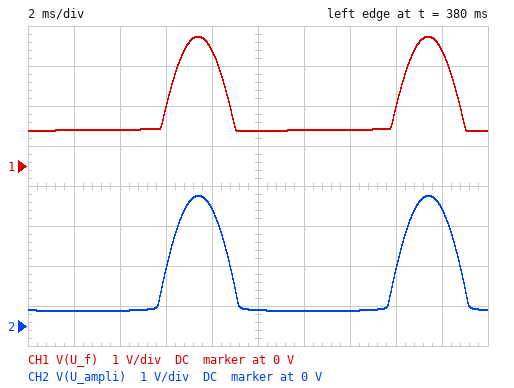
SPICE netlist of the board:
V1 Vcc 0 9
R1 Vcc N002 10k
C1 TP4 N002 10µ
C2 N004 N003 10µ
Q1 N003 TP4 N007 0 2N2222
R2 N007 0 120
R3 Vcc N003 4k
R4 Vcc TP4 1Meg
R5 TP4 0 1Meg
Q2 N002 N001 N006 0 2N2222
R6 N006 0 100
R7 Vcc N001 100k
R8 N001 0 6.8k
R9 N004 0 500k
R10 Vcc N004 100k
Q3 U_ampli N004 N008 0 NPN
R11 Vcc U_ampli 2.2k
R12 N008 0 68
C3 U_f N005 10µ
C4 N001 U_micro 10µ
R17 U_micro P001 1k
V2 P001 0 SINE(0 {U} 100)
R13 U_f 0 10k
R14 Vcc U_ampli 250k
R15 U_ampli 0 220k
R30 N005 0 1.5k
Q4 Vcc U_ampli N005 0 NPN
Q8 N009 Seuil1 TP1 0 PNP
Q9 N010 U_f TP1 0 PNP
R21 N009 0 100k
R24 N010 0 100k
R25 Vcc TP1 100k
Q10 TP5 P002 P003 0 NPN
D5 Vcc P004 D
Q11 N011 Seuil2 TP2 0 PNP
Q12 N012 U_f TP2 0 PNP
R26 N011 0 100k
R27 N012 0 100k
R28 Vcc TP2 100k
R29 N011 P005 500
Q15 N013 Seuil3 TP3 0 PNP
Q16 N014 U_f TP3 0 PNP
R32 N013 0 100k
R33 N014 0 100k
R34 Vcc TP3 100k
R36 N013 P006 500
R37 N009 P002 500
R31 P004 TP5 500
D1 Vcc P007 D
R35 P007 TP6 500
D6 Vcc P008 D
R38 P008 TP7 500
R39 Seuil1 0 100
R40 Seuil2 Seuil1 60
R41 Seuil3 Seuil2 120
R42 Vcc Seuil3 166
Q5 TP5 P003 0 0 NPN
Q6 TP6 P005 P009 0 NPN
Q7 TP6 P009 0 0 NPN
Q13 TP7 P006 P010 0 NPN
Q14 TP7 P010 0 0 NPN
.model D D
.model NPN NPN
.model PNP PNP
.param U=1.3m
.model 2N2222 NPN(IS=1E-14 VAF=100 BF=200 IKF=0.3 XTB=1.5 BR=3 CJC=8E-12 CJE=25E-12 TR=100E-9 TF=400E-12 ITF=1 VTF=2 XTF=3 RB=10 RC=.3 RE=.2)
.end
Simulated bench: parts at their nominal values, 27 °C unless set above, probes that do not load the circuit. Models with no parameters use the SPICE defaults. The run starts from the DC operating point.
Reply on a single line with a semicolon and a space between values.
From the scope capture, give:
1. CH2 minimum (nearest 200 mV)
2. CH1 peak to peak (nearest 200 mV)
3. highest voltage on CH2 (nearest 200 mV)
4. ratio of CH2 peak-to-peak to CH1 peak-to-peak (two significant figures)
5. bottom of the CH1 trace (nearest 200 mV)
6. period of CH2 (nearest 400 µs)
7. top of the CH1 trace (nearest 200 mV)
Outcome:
400 mV; 2.4 V; 3.2 V; 1.2; 800 mV; 10.0 ms; 3.2 V
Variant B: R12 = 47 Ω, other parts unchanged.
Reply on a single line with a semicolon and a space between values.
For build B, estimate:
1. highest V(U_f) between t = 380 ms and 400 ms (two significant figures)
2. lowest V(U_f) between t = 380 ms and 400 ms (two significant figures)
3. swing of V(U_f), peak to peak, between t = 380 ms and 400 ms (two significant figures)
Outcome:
3.6 V; 790 mV; 2.8 V
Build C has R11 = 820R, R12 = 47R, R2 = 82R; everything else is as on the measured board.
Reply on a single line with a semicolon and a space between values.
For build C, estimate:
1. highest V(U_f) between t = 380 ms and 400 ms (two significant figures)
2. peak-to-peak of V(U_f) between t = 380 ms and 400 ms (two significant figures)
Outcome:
4.2 V; 4.8 V
